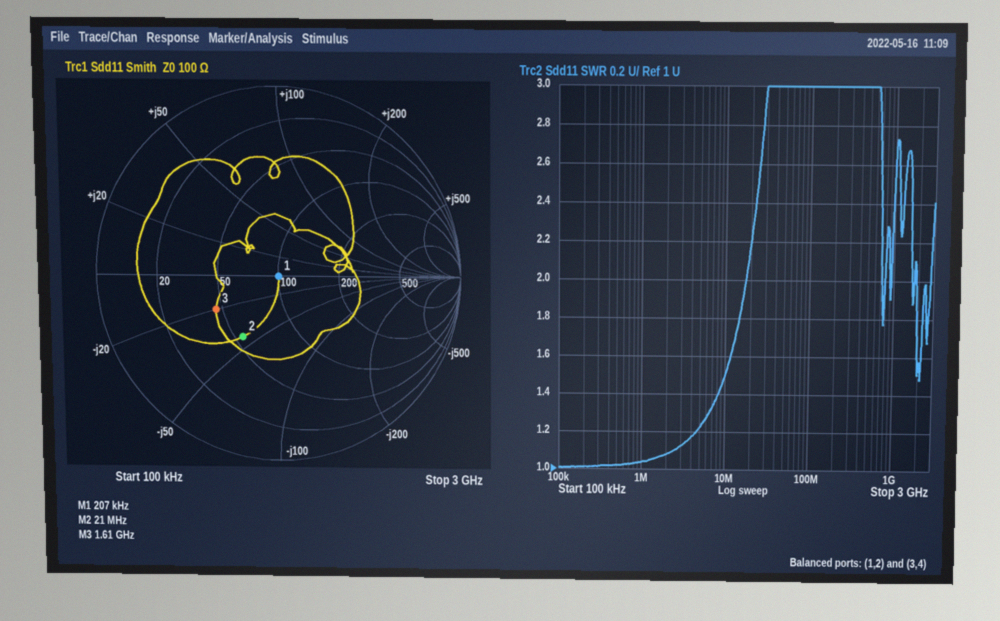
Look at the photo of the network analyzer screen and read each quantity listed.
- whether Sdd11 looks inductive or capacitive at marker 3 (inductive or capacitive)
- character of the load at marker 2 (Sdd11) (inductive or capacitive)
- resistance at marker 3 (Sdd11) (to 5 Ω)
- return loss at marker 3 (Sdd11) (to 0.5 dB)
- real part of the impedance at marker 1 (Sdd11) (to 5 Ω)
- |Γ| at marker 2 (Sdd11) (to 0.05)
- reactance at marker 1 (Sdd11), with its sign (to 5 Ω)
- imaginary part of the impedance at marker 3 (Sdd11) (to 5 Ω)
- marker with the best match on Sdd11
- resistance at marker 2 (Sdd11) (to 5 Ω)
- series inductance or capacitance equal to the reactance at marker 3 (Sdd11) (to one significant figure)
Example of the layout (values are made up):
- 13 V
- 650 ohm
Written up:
- capacitive
- capacitive
- 45 Ω
- 8.0 dB
- 100 Ω
- 0.40
- 0 Ω
- -20 Ω
- marker 1
- 55 Ω
- 5 pF
